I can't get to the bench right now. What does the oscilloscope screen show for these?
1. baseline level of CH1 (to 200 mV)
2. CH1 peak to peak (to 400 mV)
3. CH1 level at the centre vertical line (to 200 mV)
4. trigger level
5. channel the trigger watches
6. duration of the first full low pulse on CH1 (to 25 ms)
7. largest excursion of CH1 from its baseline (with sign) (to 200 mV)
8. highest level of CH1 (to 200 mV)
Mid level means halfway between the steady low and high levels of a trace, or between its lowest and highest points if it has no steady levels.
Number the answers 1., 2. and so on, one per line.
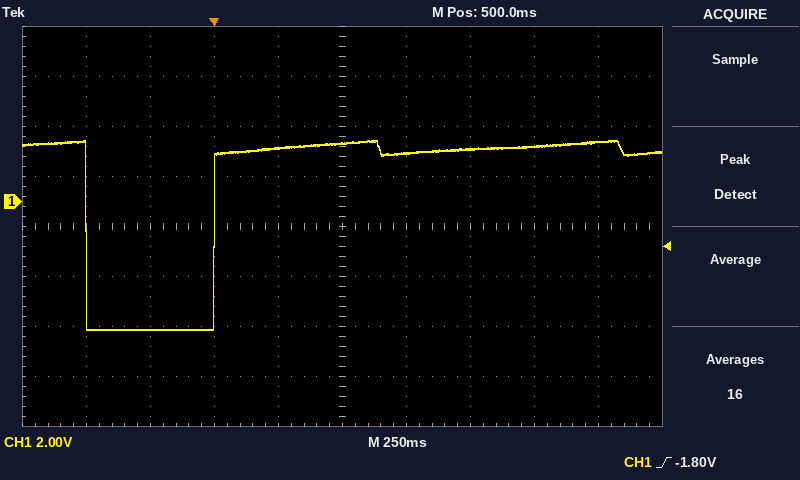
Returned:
1. 2.2 V
2. 7.6 V
3. 2.4 V
4. -1.80 V
5. CH1
6. 500 ms
7. -7.2 V
8. 2.4 V
